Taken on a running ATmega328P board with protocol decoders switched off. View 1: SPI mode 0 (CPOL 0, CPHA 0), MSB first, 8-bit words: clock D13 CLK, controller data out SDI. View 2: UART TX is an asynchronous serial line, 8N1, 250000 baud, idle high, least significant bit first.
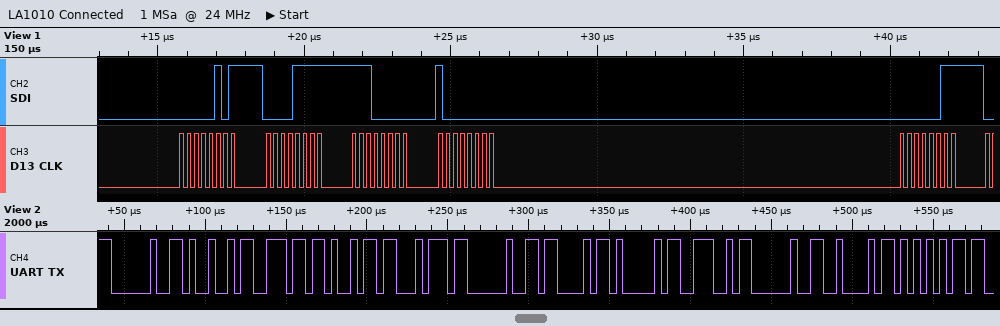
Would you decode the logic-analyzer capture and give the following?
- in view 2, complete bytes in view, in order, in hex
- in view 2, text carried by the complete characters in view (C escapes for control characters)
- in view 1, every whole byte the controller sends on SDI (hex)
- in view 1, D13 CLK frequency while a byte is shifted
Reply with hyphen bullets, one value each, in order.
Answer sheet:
- 20 49 6E 69 74 20 43 41 4E 20 42 55
- " Init CAN BU"
- 05 0F E0 80 03
- 4 MHz
